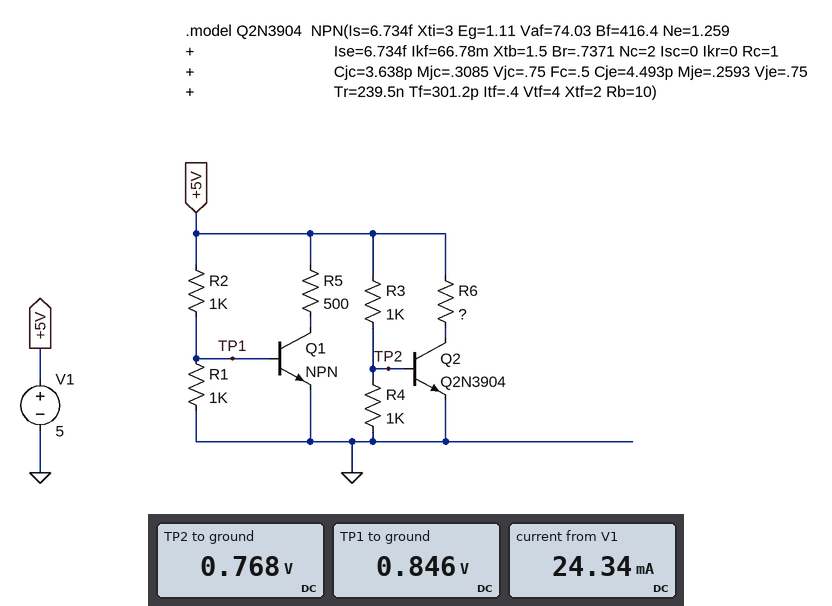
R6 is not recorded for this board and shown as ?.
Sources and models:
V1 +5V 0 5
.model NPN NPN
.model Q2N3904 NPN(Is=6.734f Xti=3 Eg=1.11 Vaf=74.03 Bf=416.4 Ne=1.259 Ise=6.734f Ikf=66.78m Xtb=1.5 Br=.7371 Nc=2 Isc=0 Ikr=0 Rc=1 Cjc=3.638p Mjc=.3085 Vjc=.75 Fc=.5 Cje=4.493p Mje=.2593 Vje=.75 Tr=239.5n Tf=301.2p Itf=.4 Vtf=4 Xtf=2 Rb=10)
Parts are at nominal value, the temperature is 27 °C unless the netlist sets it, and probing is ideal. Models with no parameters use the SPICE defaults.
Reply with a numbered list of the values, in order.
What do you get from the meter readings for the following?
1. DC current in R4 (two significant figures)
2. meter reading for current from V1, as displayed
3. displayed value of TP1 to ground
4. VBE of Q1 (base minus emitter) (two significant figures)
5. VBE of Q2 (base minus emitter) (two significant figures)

1. 770 µA
2. 24.34 mA
3. 0.846 V
4. 850 mV
5. 770 mV
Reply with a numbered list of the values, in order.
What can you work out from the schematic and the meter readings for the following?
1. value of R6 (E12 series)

1. 820 Ω
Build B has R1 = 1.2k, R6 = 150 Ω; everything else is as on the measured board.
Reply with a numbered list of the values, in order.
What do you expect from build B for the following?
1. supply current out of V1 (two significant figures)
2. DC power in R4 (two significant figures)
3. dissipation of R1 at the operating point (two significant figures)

1. 51 mA
2. 650 µW
3. 600 µW
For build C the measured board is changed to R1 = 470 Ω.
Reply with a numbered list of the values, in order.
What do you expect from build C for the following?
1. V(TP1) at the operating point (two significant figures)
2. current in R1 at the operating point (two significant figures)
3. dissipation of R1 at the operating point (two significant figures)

1. 840 mV
2. 1.8 mA
3. 1.5 mW
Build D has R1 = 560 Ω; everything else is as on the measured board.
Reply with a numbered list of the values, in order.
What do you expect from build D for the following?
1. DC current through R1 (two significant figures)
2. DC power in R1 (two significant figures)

1. 1.5 mA
2. 1.3 mW
